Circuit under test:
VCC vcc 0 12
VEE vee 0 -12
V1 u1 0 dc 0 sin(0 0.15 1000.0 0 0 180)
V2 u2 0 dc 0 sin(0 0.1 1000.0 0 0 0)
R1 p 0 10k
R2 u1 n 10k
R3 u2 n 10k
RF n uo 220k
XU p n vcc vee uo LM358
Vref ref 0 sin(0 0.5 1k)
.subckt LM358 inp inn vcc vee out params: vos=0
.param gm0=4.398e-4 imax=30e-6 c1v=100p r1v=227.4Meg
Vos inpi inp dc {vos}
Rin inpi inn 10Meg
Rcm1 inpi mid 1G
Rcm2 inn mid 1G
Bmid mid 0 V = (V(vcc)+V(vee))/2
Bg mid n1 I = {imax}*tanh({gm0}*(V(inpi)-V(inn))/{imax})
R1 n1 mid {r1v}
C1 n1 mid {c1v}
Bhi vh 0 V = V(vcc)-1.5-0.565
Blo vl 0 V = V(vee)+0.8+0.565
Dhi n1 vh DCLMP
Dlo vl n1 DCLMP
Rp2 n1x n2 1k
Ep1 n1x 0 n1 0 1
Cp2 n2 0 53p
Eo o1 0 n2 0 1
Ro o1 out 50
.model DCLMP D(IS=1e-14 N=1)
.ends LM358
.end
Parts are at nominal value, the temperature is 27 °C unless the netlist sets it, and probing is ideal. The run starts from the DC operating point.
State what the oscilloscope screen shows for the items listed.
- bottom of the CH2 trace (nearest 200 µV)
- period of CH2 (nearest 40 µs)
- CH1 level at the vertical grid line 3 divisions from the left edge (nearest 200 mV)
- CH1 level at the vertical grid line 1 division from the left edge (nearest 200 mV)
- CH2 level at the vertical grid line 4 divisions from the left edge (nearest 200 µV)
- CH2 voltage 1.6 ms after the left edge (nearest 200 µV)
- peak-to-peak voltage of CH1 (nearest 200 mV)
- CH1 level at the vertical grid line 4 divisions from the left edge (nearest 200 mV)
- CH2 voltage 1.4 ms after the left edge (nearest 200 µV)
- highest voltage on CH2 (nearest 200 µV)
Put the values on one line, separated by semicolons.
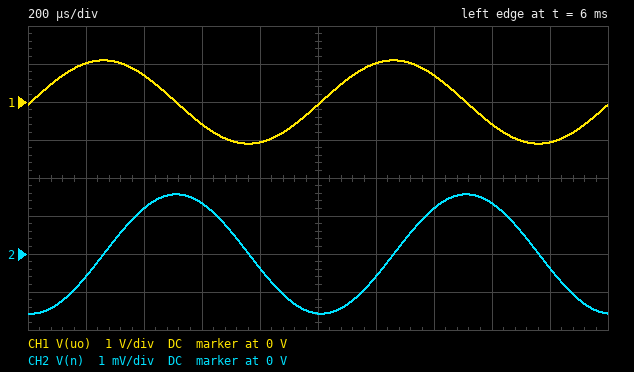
-1.6 mV; 1.00 ms; -600 mV; 1.0 V; -400 µV; 1.4 mV; 2.2 V; -1.0 V; 1.2 mV; 1.6 mV
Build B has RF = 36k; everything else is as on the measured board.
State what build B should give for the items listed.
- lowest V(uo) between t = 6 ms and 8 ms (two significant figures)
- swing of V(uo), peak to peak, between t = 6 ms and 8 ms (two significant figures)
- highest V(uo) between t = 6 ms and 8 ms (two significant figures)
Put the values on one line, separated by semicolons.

-180 mV; 360 mV; 180 mV
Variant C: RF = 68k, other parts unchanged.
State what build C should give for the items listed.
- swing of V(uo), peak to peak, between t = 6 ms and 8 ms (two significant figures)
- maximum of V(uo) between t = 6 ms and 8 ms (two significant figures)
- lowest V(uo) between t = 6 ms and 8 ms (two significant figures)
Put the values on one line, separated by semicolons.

680 mV; 340 mV; -340 mV
